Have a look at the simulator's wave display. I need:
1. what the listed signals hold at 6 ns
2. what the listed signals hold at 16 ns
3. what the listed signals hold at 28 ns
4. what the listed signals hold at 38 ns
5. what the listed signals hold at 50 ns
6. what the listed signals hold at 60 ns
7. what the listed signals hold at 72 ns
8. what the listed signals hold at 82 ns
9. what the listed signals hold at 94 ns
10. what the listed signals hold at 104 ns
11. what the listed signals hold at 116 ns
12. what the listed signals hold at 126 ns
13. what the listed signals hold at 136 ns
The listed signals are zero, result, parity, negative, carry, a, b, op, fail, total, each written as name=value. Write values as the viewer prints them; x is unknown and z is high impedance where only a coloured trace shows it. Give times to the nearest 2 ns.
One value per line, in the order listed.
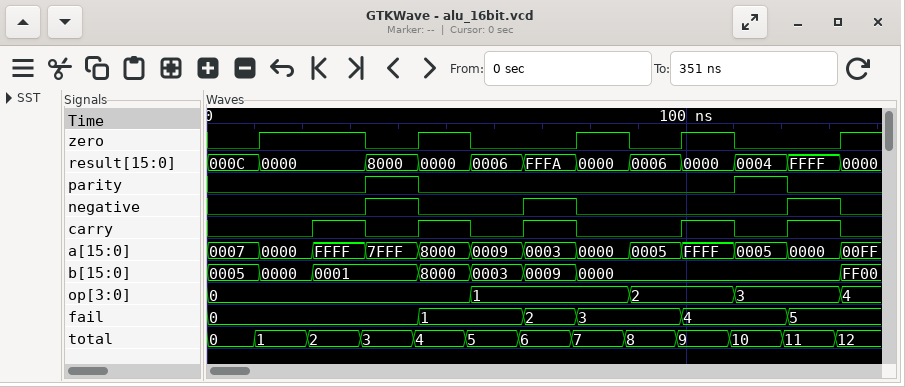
zero=0, result=000C, parity=0, negative=0, carry=0, a=0007, b=0005, op=0, fail=0, total=0
zero=1, result=0000, parity=0, negative=0, carry=0, a=0000, b=0000, op=0, fail=0, total=1
zero=1, result=0000, parity=0, negative=0, carry=1, a=FFFF, b=0001, op=0, fail=0, total=2
zero=0, result=8000, parity=1, negative=1, carry=0, a=7FFF, b=0001, op=0, fail=0, total=3
zero=1, result=0000, parity=0, negative=0, carry=1, a=8000, b=8000, op=0, fail=1, total=4
zero=0, result=0006, parity=0, negative=0, carry=0, a=0009, b=0003, op=1, fail=1, total=5
zero=0, result=FFFA, parity=0, negative=1, carry=1, a=0003, b=0009, op=1, fail=2, total=6
zero=1, result=0000, parity=0, negative=0, carry=0, a=0000, b=0000, op=1, fail=3, total=7
zero=0, result=0006, parity=0, negative=0, carry=0, a=0005, b=0000, op=2, fail=3, total=8
zero=1, result=0000, parity=0, negative=0, carry=1, a=FFFF, b=0000, op=2, fail=4, total=9
zero=0, result=0004, parity=1, negative=0, carry=0, a=0005, b=0000, op=3, fail=4, total=10
zero=0, result=FFFF, parity=0, negative=1, carry=1, a=0000, b=0000, op=3, fail=5, total=11
zero=1, result=0000, parity=0, negative=0, carry=0, a=00FF, b=FF00, op=4, fail=5, total=12
